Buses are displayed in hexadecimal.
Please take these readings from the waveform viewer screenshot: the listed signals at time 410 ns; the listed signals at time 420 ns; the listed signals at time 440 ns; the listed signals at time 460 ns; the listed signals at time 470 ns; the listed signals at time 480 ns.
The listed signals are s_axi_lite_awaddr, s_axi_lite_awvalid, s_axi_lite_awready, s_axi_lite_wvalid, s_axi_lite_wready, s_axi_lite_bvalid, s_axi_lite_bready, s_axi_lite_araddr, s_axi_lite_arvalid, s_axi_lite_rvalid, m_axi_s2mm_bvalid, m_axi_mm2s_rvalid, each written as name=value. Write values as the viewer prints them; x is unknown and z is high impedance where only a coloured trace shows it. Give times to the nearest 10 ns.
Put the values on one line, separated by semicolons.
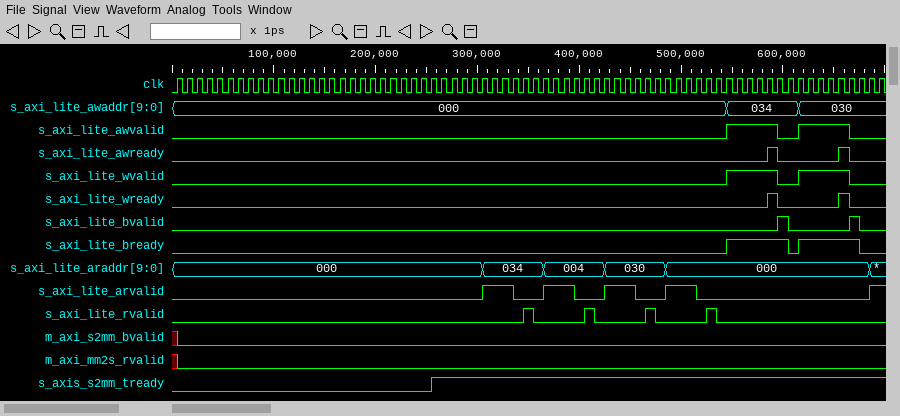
s_axi_lite_awaddr=000, s_axi_lite_awvalid=0, s_axi_lite_awready=0, s_axi_lite_wvalid=0, s_axi_lite_wready=0, s_axi_lite_bvalid=0, s_axi_lite_bready=0, s_axi_lite_araddr=004, s_axi_lite_arvalid=0, s_axi_lite_rvalid=1, m_axi_s2mm_bvalid=0, m_axi_mm2s_rvalid=0; s_axi_lite_awaddr=000, s_axi_lite_awvalid=0, s_axi_lite_awready=0, s_axi_lite_wvalid=0, s_axi_lite_wready=0, s_axi_lite_bvalid=0, s_axi_lite_bready=0, s_axi_lite_araddr=004, s_axi_lite_arvalid=0, s_axi_lite_rvalid=0, m_axi_s2mm_bvalid=0, m_axi_mm2s_rvalid=0; s_axi_lite_awaddr=000, s_axi_lite_awvalid=0, s_axi_lite_awready=0, s_axi_lite_wvalid=0, s_axi_lite_wready=0, s_axi_lite_bvalid=0, s_axi_lite_bready=0, s_axi_lite_araddr=030, s_axi_lite_arvalid=1, s_axi_lite_rvalid=0, m_axi_s2mm_bvalid=0, m_axi_mm2s_rvalid=0; s_axi_lite_awaddr=000, s_axi_lite_awvalid=0, s_axi_lite_awready=0, s_axi_lite_wvalid=0, s_axi_lite_wready=0, s_axi_lite_bvalid=0, s_axi_lite_bready=0, s_axi_lite_araddr=030, s_axi_lite_arvalid=0, s_axi_lite_rvalid=0, m_axi_s2mm_bvalid=0, m_axi_mm2s_rvalid=0; s_axi_lite_awaddr=000, s_axi_lite_awvalid=0, s_axi_lite_awready=0, s_axi_lite_wvalid=0, s_axi_lite_wready=0, s_axi_lite_bvalid=0, s_axi_lite_bready=0, s_axi_lite_araddr=030, s_axi_lite_arvalid=0, s_axi_lite_rvalid=1, m_axi_s2mm_bvalid=0, m_axi_mm2s_rvalid=0; s_axi_lite_awaddr=000, s_axi_lite_awvalid=0, s_axi_lite_awready=0, s_axi_lite_wvalid=0, s_axi_lite_wready=0, s_axi_lite_bvalid=0, s_axi_lite_bready=0, s_axi_lite_araddr=030, s_axi_lite_arvalid=0, s_axi_lite_rvalid=0, m_axi_s2mm_bvalid=0, m_axi_mm2s_rvalid=0
